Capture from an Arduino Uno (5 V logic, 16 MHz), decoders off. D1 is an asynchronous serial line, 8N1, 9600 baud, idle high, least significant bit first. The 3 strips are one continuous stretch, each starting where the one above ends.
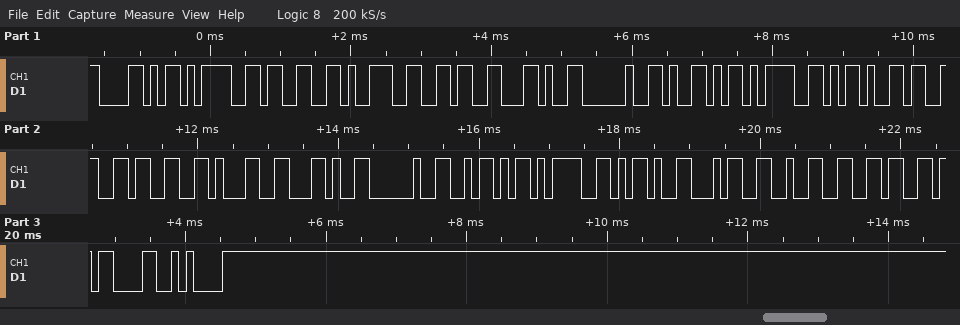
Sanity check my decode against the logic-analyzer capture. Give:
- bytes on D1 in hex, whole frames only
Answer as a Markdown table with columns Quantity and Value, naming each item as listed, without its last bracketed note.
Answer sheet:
| Quantity | Value |
|---|---|
| bytes on D1 in hex, whole frames only | 0x58 0x3D 0x33 0x39 0x36 0x2C 0x20 0x59 0x3D 0x2D 0x33 0x33 0x31 0x2C 0x20 0x5A 0x3D 0x2D 0x34 0x32 0x36 0x0D 0x0A |
